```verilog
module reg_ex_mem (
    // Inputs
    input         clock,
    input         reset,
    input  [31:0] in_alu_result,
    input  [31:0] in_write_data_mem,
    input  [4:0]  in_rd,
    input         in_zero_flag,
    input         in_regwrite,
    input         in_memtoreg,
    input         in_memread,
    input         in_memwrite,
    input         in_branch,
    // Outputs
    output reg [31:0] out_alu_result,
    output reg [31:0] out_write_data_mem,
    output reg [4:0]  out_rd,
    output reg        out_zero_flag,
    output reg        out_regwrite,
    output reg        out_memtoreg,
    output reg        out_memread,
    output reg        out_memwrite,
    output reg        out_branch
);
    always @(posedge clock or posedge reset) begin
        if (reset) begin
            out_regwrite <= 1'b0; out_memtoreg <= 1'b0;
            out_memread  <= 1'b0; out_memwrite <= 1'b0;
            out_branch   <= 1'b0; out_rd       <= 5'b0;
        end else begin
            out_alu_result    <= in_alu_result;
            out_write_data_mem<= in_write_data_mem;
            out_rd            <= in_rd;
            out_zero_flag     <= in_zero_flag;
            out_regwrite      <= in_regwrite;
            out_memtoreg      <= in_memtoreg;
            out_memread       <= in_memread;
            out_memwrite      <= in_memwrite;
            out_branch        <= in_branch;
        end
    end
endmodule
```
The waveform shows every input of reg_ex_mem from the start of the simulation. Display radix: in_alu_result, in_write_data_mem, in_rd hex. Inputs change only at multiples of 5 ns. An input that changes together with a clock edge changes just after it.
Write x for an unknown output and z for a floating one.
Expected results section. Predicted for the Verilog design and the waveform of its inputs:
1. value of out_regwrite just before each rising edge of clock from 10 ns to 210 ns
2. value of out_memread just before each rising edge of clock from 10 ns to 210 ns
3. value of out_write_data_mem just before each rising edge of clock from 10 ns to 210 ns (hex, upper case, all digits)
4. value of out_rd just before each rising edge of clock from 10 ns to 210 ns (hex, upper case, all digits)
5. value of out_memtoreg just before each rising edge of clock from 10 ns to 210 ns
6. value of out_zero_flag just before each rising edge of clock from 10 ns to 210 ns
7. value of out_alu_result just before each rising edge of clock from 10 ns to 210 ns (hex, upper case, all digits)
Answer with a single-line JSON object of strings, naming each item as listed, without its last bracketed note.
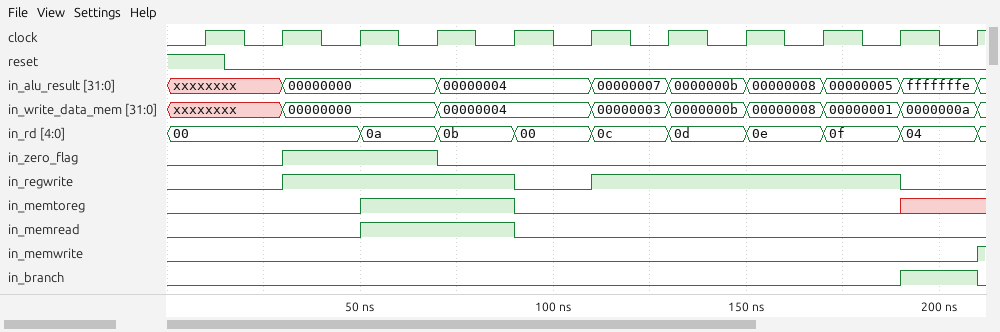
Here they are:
{"value of out_regwrite just before each rising edge of clock from 10 ns to 210 ns": "0 0 0 1 1 1 0 1 1 1 1", "value of out_memread just before each rising edge of clock from 10 ns to 210 ns": "0 0 0 0 1 1 0 0 0 0 0", "value of out_write_data_mem just before each rising edge of clock from 10 ns to 210 ns": "x, x, x, 00000000, 00000000, 00000004, 00000004, 00000003, 0000000B, 00000008, 00000001", "value of out_rd just before each rising edge of clock from 10 ns to 210 ns": "00, 00, 00, 00, 0A, 0B, 00, 0C, 0D, 0E, 0F", "value of out_memtoreg just before each rising edge of clock from 10 ns to 210 ns": "0 0 0 0 1 1 0 0 0 0 0", "value of out_zero_flag just before each rising edge of clock from 10 ns to 210 ns": "x x 0 1 1 0 0 0 0 0 0", "value of out_alu_result just before each rising edge of clock from 10 ns to 210 ns": "x, x, x, 00000000, 00000000, 00000004, 00000004, 00000007, 0000000B, 00000008, 00000005"}
